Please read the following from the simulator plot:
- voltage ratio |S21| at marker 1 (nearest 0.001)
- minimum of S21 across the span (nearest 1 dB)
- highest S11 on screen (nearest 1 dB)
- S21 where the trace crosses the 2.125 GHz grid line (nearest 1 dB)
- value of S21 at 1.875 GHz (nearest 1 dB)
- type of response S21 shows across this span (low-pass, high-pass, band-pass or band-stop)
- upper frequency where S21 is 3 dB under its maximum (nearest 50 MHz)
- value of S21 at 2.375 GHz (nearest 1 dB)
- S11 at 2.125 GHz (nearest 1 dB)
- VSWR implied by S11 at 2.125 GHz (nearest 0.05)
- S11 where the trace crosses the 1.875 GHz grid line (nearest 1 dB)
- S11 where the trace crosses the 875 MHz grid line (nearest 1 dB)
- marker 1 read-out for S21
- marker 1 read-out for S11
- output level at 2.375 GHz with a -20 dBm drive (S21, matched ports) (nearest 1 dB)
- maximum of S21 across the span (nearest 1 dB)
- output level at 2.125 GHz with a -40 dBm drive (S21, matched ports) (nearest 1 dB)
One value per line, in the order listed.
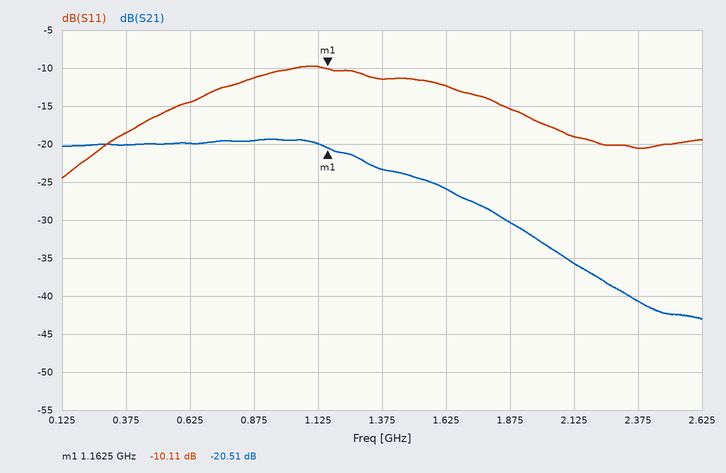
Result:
0.094
-43 dB
-10 dB
-36 dB
-30 dB
low-pass
1.30 GHz
-41 dB
-19 dB
1.25
-15 dB
-11 dB
-20.51 dB
-10.11 dB
-61 dBm
-19 dB
-76 dBm
